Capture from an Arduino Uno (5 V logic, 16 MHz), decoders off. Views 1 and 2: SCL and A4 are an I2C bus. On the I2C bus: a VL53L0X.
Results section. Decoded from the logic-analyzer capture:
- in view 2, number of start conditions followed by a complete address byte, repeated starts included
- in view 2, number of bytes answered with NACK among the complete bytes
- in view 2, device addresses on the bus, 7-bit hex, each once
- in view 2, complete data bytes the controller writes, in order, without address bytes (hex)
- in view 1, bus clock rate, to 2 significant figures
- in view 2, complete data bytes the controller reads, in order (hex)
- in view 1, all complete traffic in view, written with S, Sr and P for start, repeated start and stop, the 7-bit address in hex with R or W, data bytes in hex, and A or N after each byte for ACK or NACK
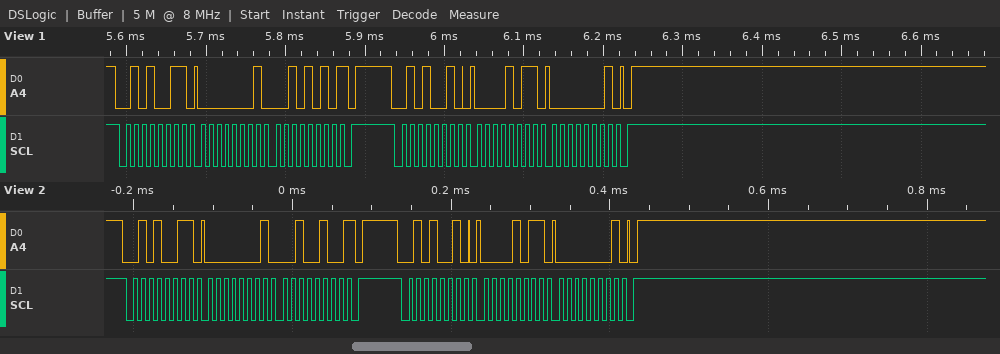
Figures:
2
1
0x29
0B 01
100 kHz
01 24
S 29R A 01 A 2A N P S 29W A 0B A 01 A P
